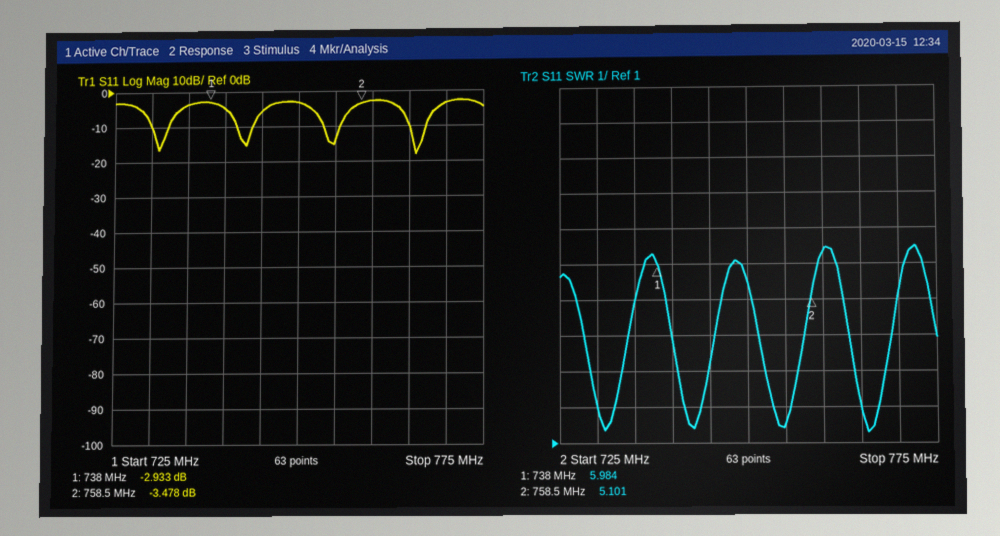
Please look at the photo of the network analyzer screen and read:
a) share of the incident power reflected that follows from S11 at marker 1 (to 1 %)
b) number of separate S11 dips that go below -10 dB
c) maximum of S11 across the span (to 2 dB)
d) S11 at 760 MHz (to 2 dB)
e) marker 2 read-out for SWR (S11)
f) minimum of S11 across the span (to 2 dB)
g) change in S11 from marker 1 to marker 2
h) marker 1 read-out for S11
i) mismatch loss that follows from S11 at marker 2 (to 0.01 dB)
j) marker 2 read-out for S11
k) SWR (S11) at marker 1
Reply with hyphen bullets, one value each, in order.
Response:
- 51 %
- 4
- -2 dB
- -2 dB
- 5.101
- -18 dB
- -0.545 dB
- -2.933 dB
- 2.59 dB
- -3.478 dB
- 5.984
